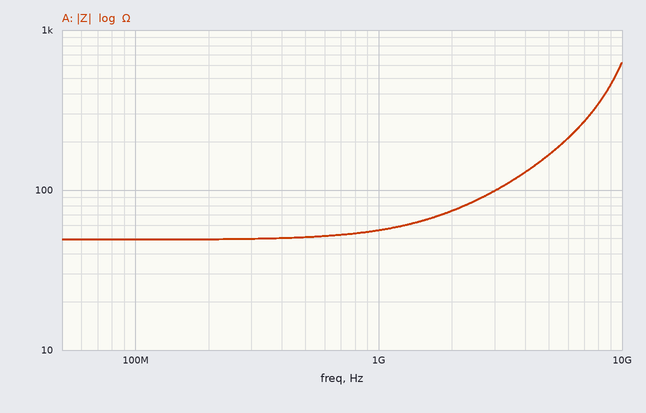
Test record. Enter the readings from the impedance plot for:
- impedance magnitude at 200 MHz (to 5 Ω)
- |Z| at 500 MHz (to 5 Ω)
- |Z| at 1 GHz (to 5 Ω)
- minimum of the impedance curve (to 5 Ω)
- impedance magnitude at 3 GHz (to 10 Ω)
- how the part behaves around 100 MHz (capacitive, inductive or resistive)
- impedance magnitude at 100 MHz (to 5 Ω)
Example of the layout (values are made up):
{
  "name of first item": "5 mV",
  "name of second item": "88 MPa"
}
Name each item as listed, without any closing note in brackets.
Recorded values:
{
  "impedance magnitude at 200 MHz": "50 Ω",
  "|Z| at 500 MHz": "50 Ω",
  "|Z| at 1 GHz": "55 Ω",
  "minimum of the impedance curve": "50 Ω",
  "impedance magnitude at 3 GHz": "100 Ω",
  "how the part behaves around 100 MHz": "resistive",
  "impedance magnitude at 100 MHz": "50 Ω"
}
